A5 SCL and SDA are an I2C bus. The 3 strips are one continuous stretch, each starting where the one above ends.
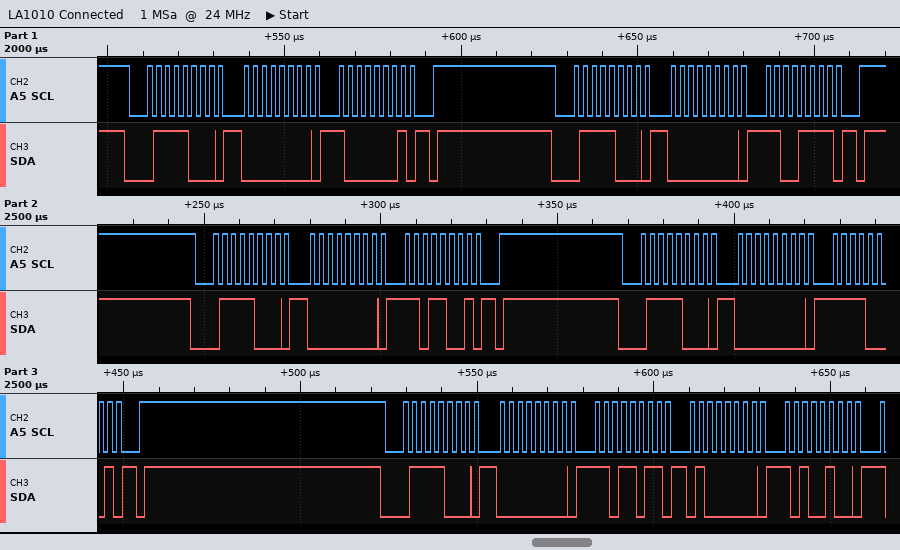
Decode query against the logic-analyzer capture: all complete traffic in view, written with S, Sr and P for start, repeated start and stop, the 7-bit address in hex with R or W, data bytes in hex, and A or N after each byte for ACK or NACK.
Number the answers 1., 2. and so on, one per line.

1. S 3CW A 00 A 81 A P S 3CW A 00 A CF A P S 3CW A 00 A D9 A P S 3CW A 00 A F1 A P S 3CW A 00 A DB A 40 A A4 A
